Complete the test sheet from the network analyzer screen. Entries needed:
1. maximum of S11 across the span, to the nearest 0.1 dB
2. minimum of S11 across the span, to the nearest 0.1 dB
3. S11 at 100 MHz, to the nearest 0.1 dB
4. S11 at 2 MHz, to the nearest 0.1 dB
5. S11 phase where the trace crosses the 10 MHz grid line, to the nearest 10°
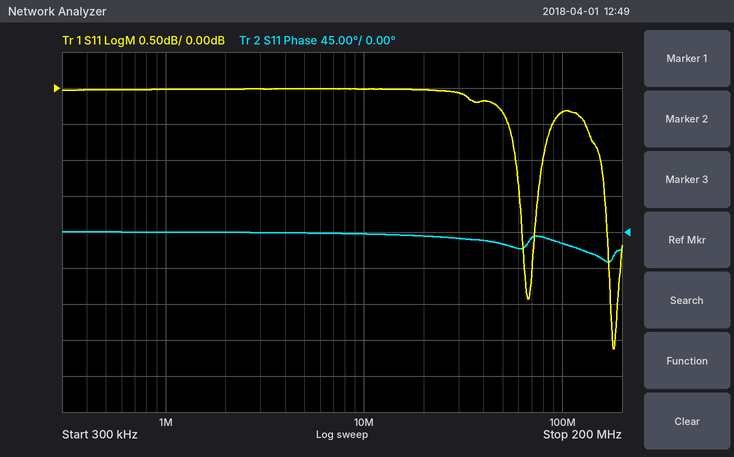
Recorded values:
0.0 dB
-3.6 dB
-0.3 dB
0.0 dB
0°
